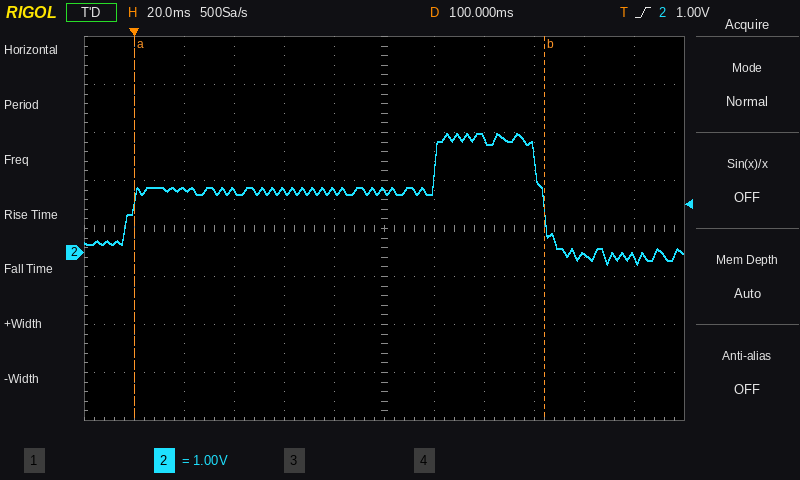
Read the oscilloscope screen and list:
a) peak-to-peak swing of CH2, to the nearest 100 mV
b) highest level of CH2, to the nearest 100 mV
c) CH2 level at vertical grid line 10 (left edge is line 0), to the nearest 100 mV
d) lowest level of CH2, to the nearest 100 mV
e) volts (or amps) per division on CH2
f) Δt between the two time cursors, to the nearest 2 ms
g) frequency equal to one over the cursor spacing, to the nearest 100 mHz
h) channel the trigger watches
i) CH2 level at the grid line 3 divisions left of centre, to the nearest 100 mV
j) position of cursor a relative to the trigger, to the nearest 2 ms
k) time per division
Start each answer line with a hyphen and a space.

- 2.7 V
- 2.5 V
- 0.0 V
- -200 mV
- 1 V
- 164 ms
- 6.1 Hz
- CH2
- 1.3 V
- 0 ms
- 20 ms
